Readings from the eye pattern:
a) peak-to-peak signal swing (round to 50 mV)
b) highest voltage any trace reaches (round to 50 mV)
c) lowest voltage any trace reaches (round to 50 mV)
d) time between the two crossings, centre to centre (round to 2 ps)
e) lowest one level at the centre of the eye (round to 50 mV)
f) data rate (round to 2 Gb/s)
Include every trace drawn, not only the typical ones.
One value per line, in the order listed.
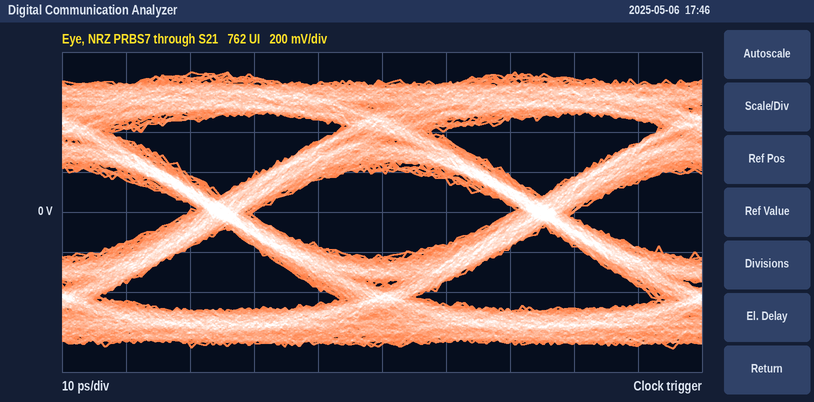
1.40 V
700 mV
-700 mV
50 ps
200 mV
20 Gb/s
